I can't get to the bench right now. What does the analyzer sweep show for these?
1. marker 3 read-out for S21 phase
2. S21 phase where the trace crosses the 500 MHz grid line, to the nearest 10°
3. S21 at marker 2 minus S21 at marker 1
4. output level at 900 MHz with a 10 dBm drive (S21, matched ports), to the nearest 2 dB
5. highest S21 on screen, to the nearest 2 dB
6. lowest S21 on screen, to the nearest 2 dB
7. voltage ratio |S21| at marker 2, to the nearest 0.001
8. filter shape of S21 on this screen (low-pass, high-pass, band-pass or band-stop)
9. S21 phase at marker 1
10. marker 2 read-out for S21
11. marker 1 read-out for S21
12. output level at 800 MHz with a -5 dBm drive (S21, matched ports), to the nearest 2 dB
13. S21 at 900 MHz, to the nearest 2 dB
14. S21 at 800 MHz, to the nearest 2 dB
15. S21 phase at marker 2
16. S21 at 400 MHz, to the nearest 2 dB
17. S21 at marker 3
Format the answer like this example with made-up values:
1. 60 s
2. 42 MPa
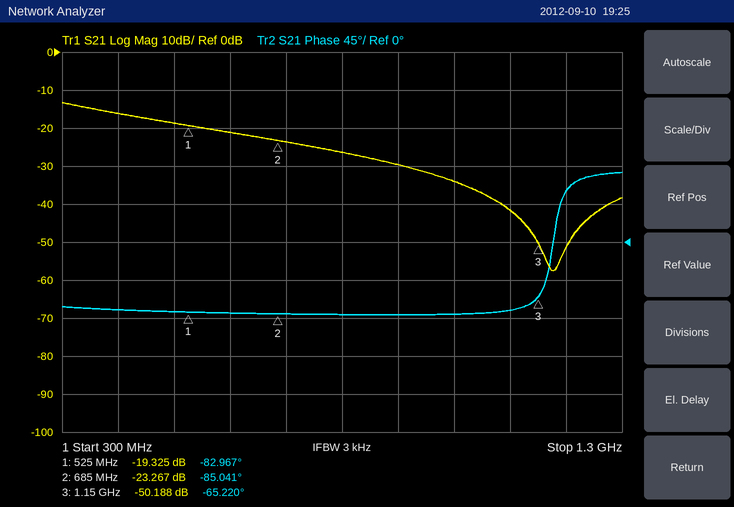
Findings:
1. -65.220°
2. -80°
3. -3.942 dB
4. -20 dBm
5. -14 dB
6. -58 dB
7. 0.069
8. low-pass
9. -82.967°
10. -23.267 dB
11. -19.325 dB
12. -32 dBm
13. -30 dB
14. -26 dB
15. -85.041°
16. -16 dB
17. -50.188 dB
